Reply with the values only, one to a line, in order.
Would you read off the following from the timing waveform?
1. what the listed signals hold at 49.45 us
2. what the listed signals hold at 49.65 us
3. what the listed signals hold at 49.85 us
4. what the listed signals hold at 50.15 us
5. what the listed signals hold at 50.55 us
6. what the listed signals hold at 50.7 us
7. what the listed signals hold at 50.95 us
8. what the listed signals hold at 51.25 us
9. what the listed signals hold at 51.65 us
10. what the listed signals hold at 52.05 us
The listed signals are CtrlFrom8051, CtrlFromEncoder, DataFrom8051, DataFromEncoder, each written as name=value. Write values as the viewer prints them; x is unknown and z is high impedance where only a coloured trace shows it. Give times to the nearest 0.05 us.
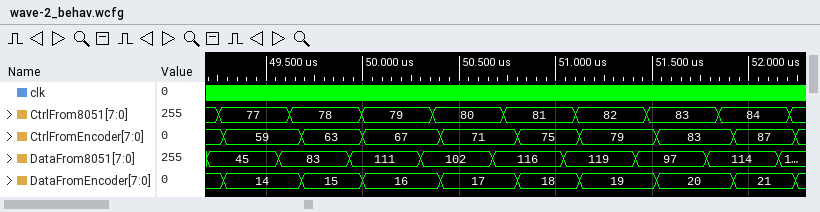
CtrlFrom8051=77, CtrlFromEncoder=59, DataFrom8051=45, DataFromEncoder=14
CtrlFrom8051=78, CtrlFromEncoder=59, DataFrom8051=83, DataFromEncoder=14
CtrlFrom8051=78, CtrlFromEncoder=63, DataFrom8051=83, DataFromEncoder=15
CtrlFrom8051=79, CtrlFromEncoder=67, DataFrom8051=111, DataFromEncoder=16
CtrlFrom8051=80, CtrlFromEncoder=71, DataFrom8051=102, DataFromEncoder=17
CtrlFrom8051=80, CtrlFromEncoder=71, DataFrom8051=116, DataFromEncoder=17
CtrlFrom8051=81, CtrlFromEncoder=75, DataFrom8051=116, DataFromEncoder=18
CtrlFrom8051=82, CtrlFromEncoder=79, DataFrom8051=119, DataFromEncoder=19
CtrlFrom8051=83, CtrlFromEncoder=83, DataFrom8051=97, DataFromEncoder=20
CtrlFrom8051=84, CtrlFromEncoder=87, DataFrom8051=114, DataFromEncoder=21
